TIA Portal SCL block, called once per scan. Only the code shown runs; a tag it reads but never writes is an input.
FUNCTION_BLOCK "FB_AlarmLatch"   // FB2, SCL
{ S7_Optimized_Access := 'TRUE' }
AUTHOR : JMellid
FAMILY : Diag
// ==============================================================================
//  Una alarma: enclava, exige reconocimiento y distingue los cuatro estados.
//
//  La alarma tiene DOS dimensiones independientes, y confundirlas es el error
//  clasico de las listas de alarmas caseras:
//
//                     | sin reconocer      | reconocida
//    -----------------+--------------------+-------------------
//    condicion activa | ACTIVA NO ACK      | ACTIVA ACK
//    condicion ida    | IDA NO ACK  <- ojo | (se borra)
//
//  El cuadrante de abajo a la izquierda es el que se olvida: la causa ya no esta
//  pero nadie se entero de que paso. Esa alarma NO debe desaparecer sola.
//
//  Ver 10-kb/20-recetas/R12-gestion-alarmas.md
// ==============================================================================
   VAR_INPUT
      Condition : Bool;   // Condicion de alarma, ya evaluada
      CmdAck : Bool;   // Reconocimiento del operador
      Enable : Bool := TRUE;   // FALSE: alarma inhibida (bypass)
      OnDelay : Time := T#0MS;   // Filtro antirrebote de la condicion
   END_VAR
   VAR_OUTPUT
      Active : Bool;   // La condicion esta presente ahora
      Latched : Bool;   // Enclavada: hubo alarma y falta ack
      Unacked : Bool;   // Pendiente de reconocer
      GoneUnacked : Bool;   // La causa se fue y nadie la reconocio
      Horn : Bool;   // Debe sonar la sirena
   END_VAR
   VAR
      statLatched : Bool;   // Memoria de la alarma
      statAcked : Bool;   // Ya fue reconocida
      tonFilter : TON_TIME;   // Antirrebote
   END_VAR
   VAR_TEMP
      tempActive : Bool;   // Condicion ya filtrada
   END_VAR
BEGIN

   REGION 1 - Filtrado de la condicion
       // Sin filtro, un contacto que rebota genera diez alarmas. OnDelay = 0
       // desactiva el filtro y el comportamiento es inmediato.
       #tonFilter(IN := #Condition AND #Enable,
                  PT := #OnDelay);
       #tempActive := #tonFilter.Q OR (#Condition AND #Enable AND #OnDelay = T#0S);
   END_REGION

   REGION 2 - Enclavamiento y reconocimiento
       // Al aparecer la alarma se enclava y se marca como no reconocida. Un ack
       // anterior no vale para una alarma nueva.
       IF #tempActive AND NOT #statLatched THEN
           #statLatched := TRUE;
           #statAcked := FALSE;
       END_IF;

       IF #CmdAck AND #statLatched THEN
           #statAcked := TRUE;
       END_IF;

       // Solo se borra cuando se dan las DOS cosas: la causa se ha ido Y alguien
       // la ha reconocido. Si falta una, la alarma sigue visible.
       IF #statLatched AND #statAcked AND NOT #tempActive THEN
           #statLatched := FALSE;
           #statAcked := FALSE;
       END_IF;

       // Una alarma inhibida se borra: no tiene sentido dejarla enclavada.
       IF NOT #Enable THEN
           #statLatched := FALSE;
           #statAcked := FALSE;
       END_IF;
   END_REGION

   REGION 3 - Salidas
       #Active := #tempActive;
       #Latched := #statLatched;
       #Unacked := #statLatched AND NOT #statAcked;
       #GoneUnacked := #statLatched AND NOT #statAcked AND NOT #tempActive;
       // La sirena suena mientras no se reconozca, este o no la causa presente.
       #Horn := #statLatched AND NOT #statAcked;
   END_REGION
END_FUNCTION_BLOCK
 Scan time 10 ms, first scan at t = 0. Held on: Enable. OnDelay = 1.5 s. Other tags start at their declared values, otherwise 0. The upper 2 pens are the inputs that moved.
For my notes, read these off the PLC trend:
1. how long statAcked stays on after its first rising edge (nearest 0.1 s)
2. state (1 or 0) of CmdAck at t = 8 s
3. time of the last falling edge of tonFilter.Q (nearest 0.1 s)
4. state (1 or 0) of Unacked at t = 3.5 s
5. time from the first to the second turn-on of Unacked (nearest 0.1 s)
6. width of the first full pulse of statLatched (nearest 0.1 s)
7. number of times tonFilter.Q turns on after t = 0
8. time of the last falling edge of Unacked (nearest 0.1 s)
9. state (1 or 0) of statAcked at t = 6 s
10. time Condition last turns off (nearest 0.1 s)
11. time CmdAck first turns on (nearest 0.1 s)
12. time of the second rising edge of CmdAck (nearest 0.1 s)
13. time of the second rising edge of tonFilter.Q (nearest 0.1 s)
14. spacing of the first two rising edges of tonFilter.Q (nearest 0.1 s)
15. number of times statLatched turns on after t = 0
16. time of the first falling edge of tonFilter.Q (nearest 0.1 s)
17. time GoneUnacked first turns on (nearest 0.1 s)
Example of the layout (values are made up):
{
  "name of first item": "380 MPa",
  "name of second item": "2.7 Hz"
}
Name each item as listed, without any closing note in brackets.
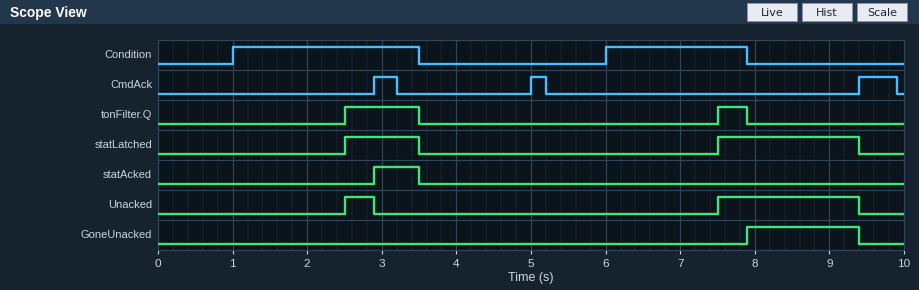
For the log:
{
  "how long statAcked stays on after its first rising edge": "0.6 s",
  "state (1 or 0) of CmdAck at t = 8 s": "0",
  "time of the last falling edge of tonFilter.Q": "7.9 s",
  "state (1 or 0) of Unacked at t = 3.5 s": "0",
  "time from the first to the second turn-on of Unacked": "5.0 s",
  "width of the first full pulse of statLatched": "1.0 s",
  "number of times tonFilter.Q turns on after t = 0": "2",
  "time of the last falling edge of Unacked": "9.4 s",
  "state (1 or 0) of statAcked at t = 6 s": "0",
  "time Condition last turns off": "7.9 s",
  "time CmdAck first turns on": "2.9 s",
  "time of the second rising edge of CmdAck": "5.0 s",
  "time of the second rising edge of tonFilter.Q": "7.5 s",
  "spacing of the first two rising edges of tonFilter.Q": "5.0 s",
  "number of times statLatched turns on after t = 0": "2",
  "time of the first falling edge of tonFilter.Q": "3.5 s",
  "time GoneUnacked first turns on": "7.9 s"
}
